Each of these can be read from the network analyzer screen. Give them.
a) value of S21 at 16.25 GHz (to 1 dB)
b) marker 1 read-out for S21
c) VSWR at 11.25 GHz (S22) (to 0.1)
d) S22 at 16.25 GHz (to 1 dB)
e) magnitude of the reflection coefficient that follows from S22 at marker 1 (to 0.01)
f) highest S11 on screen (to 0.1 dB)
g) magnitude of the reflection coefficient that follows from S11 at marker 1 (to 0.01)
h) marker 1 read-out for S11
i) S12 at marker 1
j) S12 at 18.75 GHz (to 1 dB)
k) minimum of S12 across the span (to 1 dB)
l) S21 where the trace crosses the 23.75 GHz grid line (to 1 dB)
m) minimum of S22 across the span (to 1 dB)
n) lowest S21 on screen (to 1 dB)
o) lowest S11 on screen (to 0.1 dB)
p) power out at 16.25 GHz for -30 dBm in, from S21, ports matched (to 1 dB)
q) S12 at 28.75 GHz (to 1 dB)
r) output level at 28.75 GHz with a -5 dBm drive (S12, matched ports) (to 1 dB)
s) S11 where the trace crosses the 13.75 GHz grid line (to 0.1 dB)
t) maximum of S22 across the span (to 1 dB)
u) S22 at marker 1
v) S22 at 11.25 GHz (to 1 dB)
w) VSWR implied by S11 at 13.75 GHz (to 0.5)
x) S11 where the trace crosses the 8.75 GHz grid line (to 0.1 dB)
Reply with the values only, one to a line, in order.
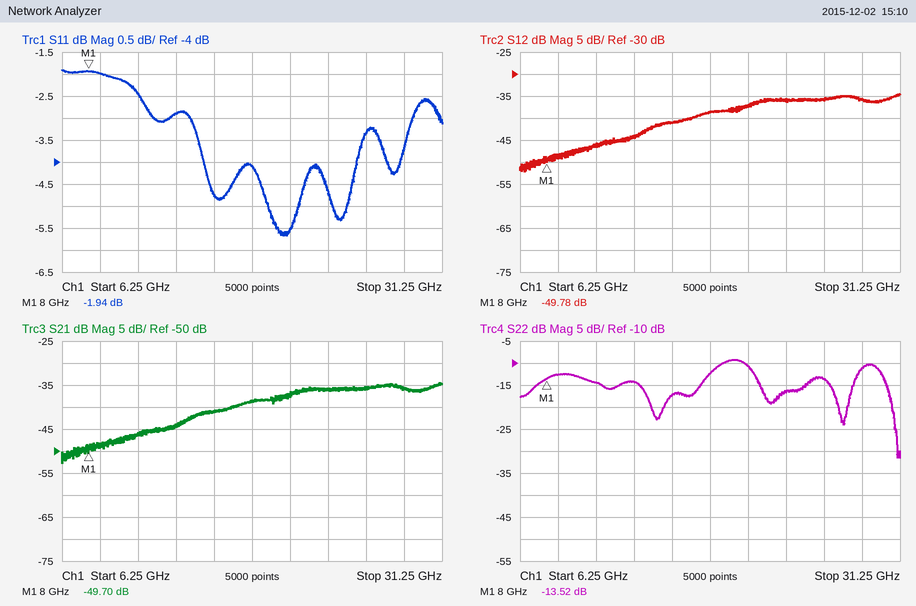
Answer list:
-41 dB
-49.70 dB
1.5
-17 dB
0.21
-1.9 dB
0.80
-1.94 dB
-49.78 dB
-39 dB
-52 dB
-36 dB
-32 dB
-53 dB
-5.7 dB
-71 dBm
-36 dB
-41 dBm
-2.9 dB
-9 dB
-13.52 dB
-14 dB
6.0
-2.0 dB
